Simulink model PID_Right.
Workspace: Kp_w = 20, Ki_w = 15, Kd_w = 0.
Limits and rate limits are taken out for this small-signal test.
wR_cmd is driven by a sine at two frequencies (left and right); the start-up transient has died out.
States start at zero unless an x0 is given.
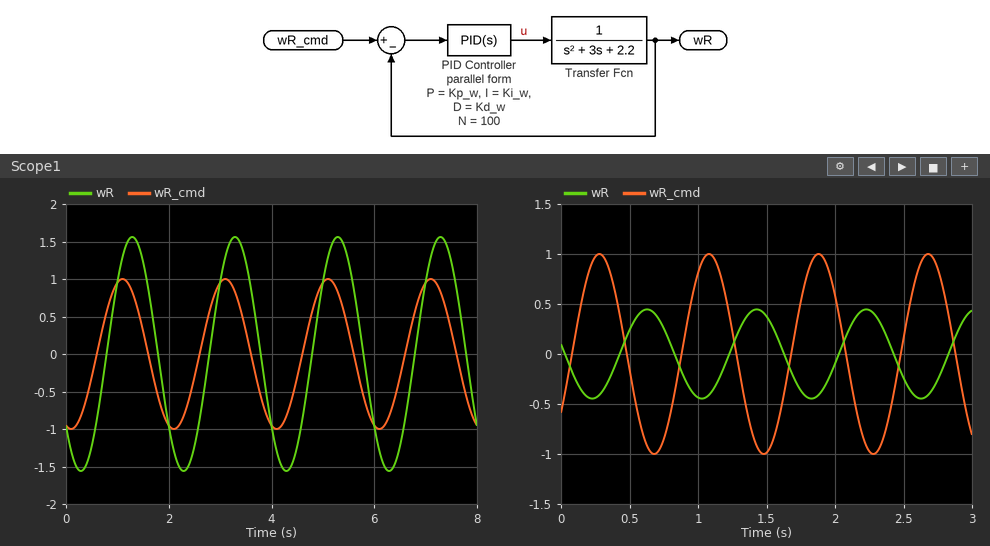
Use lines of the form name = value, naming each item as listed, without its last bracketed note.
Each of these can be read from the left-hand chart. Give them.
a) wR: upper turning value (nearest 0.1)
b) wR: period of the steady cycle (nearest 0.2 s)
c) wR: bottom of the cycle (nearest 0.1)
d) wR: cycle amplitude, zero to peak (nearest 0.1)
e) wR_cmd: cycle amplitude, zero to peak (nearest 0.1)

wR: upper turning value = 1.6
wR: period of the steady cycle = 2.0 s
wR: bottom of the cycle = -1.6
wR: cycle amplitude, zero to peak = 1.6
wR_cmd: cycle amplitude, zero to peak = 1.0
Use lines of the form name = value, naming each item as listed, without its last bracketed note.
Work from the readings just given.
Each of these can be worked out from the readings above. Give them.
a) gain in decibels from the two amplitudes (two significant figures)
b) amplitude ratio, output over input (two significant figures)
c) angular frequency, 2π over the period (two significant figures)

gain in decibels from the two amplitudes = 4.1 dB
amplitude ratio, output over input = 1.6
angular frequency, 2π over the period = 3.1 rad/s
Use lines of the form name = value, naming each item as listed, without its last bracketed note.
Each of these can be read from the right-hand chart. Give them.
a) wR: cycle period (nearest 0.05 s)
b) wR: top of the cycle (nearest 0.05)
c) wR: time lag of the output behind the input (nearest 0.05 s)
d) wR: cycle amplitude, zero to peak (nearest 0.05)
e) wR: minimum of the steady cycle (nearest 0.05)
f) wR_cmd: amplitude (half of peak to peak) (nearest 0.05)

wR: cycle period = 0.80 s
wR: top of the cycle = 0.45
wR: time lag of the output behind the input = 0.35 s
wR: cycle amplitude, zero to peak = 0.45
wR: minimum of the steady cycle = -0.45
wR_cmd: amplitude (half of peak to peak) = 1.00
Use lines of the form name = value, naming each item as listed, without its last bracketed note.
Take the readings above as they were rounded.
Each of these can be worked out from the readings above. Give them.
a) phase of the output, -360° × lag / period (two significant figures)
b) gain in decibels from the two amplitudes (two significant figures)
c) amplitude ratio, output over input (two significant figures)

phase of the output, -360° × lag / period = -160°
gain in decibels from the two amplitudes = -6.9 dB
amplitude ratio, output over input = 0.45
